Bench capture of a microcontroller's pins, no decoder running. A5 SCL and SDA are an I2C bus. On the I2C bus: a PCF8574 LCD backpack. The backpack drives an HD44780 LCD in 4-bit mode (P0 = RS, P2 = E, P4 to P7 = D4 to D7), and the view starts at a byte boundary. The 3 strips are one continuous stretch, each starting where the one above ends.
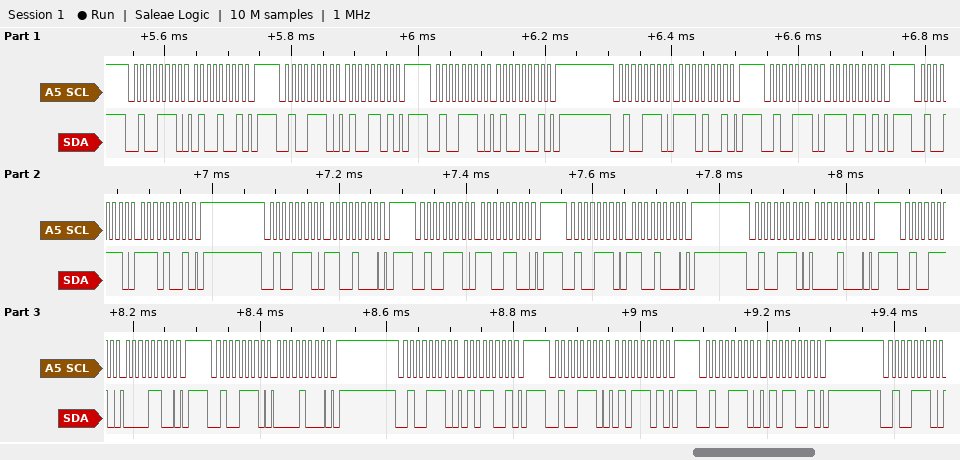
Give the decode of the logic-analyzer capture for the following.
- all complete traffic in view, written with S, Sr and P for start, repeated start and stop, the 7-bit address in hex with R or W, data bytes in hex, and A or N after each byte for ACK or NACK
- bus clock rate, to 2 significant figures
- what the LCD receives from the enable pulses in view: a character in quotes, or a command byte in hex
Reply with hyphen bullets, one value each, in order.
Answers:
- S 27W A 49 A P S 27W A 4D A P S 27W A 49 A P S 27W A E9 A P S 27W A ED A P S 27W A E9 A P S 27W A C8 A P S 27W A CC A P S 27W A C8 A P S 27W A 08 A P S 27W A 0C A P S 27W A 08 A P S 27W A 59 A P S 27W A 5D A P S 27W A 59 A P S 27W A
- 100 kHz
- 'N' 0xC0
